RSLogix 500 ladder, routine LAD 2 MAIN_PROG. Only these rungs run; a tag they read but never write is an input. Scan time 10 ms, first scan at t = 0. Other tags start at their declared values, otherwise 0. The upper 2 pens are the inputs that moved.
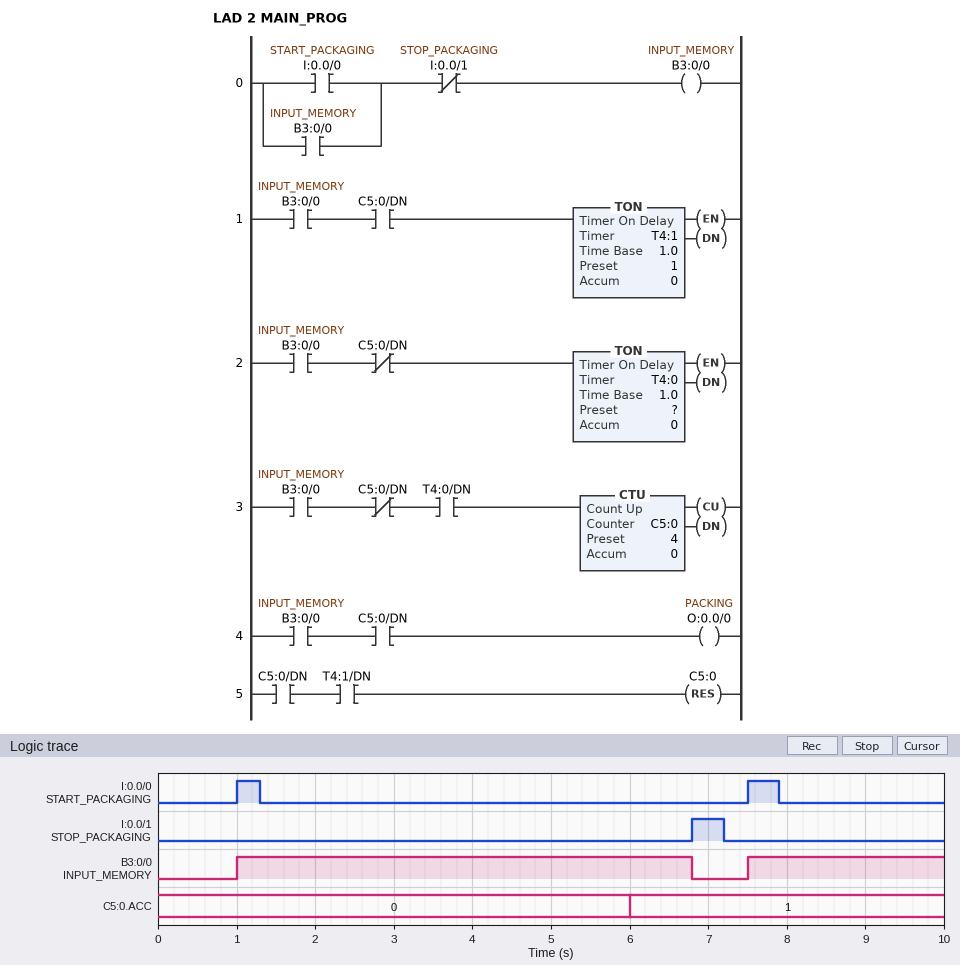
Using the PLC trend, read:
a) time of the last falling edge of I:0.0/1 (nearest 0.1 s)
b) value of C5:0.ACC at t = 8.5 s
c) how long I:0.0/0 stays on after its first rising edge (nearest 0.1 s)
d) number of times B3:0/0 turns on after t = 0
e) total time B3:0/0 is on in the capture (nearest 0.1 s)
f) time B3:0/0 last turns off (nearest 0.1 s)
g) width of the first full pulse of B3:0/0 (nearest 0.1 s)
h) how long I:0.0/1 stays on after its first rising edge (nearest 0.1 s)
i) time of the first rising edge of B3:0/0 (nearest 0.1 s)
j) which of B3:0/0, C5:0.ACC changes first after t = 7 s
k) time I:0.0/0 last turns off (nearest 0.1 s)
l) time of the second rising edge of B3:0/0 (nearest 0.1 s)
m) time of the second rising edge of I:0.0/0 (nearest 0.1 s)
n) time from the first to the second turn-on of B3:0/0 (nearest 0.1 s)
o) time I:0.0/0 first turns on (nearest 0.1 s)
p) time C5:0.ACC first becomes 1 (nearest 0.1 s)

7.2 s
1
0.3 s
2
8.3 s
6.8 s
5.8 s
0.4 s
1.0 s
B3:0/0
7.9 s
7.5 s
7.5 s
6.5 s
1.0 s
6.0 s
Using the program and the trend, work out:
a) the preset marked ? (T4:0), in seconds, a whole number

5 s
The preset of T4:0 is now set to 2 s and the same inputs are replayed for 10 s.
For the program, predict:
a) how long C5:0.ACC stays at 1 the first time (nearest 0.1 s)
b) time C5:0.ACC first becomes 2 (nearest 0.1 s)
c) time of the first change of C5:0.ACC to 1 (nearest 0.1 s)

6.5 s
9.5 s
3.0 s
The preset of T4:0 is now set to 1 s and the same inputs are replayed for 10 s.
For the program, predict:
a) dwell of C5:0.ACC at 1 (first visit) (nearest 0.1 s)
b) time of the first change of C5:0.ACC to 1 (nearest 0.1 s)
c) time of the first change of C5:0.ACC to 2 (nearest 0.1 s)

6.5 s
2.0 s
8.5 s
